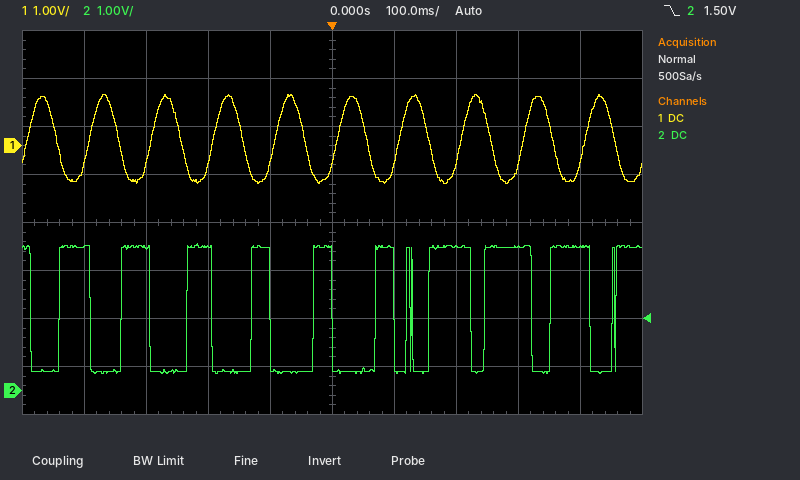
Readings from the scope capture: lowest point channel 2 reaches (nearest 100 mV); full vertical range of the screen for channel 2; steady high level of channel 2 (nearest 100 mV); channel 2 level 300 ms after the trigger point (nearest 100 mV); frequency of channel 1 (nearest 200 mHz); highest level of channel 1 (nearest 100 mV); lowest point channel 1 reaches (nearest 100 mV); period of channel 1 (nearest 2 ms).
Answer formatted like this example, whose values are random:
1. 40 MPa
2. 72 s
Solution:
1. 400 mV
2. 8 V
3. 3.0 V
4. 3.0 V
5. 10.0 Hz
6. 1.1 V
7. -800 mV
8. 100 ms
